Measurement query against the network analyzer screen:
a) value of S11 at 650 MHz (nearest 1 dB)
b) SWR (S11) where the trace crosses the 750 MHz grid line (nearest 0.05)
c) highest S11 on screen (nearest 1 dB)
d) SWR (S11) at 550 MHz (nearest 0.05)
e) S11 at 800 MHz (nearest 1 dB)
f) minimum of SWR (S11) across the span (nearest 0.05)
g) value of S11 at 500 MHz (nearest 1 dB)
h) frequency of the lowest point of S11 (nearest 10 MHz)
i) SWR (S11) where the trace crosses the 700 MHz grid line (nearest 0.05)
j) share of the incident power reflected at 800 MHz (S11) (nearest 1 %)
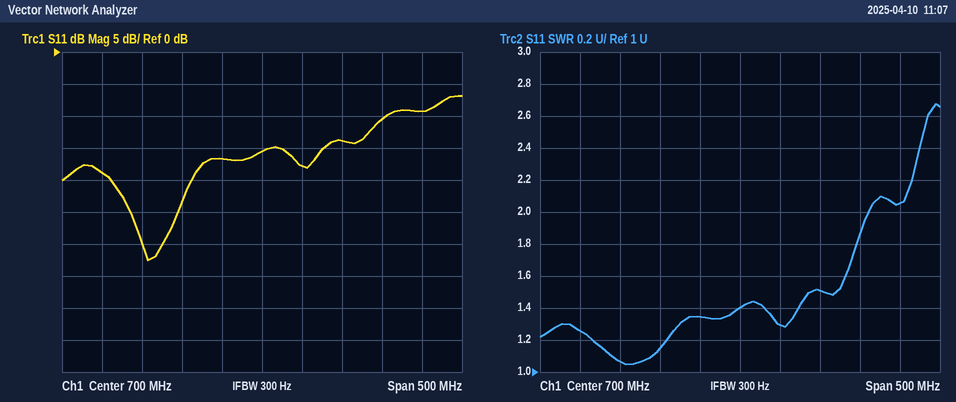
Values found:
-17 dB
1.30
-7 dB
1.05
-14 dB
1.05
-19 dB
560 MHz
1.40
4 %
